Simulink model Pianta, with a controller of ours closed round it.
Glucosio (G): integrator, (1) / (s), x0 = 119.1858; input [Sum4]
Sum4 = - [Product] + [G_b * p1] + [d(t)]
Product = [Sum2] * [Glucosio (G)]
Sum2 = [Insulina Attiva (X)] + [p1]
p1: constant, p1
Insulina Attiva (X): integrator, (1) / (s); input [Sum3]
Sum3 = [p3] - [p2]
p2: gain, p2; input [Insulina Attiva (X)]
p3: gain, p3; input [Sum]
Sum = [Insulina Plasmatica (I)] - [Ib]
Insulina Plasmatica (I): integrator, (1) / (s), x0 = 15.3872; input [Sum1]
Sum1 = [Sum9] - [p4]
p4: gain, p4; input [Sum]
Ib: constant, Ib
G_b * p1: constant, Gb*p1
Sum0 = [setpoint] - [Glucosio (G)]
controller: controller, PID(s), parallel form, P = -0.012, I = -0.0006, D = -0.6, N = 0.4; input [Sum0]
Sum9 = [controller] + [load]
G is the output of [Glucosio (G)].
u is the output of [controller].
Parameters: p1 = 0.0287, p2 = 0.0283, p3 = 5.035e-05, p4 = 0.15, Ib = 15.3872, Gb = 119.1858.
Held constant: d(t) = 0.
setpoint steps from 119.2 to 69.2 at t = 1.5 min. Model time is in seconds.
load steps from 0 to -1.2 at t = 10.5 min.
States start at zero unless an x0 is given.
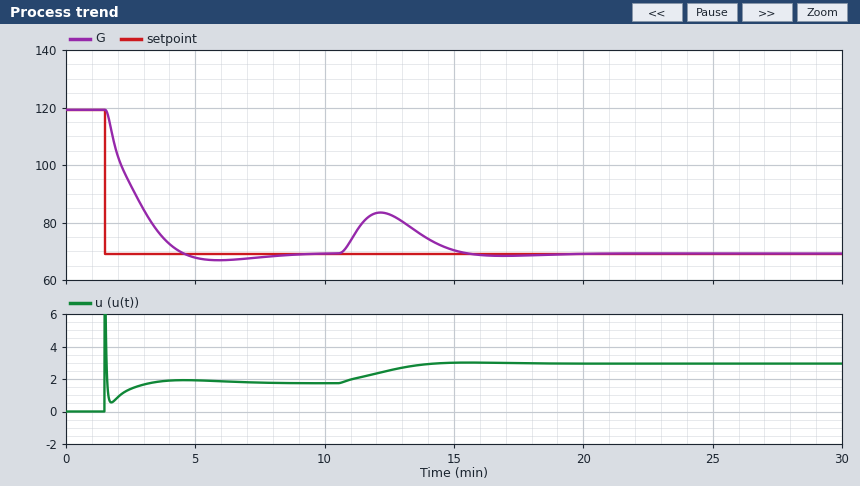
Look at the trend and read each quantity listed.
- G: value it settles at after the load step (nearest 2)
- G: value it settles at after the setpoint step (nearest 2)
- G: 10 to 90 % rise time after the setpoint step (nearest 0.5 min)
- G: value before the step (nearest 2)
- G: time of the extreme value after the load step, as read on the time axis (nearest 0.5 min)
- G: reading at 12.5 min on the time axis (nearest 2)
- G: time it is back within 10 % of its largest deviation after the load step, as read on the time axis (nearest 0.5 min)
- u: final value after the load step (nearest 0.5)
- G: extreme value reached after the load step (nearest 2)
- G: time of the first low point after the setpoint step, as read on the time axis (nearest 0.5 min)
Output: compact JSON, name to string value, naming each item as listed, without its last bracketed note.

{"G: value it settles at after the load step": "70", "G: value it settles at after the setpoint step": "70", "G: 10 to 90 % rise time after the setpoint step": "2.0 min", "G: value before the step": "120", "G: time of the extreme value after the load step, as read on the time axis": "12.0 min", "G: reading at 12.5 min on the time axis": "82", "G: time it is back within 10 % of its largest deviation after the load step, as read on the time axis": "15.0 min", "u: final value after the load step": "3.0", "G: extreme value reached after the load step": "84", "G: time of the first low point after the setpoint step, as read on the time axis": "6.0 min"}
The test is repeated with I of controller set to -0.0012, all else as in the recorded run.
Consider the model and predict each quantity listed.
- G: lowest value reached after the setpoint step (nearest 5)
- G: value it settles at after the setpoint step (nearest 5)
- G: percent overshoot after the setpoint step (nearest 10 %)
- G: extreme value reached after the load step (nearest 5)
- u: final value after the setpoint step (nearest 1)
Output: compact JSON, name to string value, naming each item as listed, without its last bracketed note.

{"G: lowest value reached after the setpoint step": "60", "G: value it settles at after the setpoint step": "70", "G: percent overshoot after the setpoint step": "20 %", "G: extreme value reached after the load step": "80", "u: final value after the setpoint step": "2"}
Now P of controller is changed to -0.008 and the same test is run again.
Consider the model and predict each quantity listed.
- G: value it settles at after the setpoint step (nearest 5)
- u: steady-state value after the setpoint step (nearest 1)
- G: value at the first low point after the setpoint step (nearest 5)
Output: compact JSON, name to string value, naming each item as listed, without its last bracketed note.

{"G: value it settles at after the setpoint step": "70", "u: steady-state value after the setpoint step": "2", "G: value at the first low point after the setpoint step": "65"}
